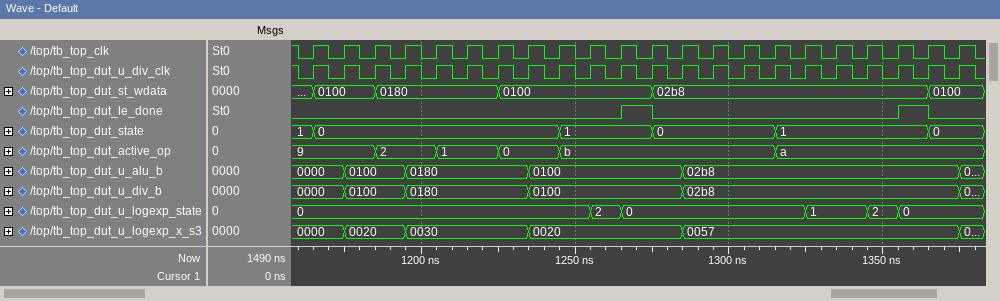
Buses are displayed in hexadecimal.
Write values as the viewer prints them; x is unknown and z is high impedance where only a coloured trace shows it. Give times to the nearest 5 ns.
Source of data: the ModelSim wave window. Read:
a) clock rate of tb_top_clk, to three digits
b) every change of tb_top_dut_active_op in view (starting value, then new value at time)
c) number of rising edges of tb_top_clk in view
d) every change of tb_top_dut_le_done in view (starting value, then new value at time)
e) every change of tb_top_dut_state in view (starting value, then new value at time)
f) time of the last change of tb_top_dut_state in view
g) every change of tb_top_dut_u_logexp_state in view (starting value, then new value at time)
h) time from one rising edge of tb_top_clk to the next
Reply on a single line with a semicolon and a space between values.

100 MHz; 9, 2 at 1185 ns, 1 at 1205 ns, 0 at 1225 ns, b at 1245 ns, a at 1315 ns; 22; 0, 1 at 1265 ns, 0 at 1275 ns, 1 at 1355 ns, 0 at 1365 ns; 1, 0 at 1165 ns, 1 at 1245 ns, 0 at 1275 ns, 1 at 1315 ns, 0 at 1365 ns; 1365 ns; 0, 2 at 1255 ns, 0 at 1265 ns, 1 at 1325 ns, 2 at 1345 ns, 0 at 1355 ns; 10 ns
